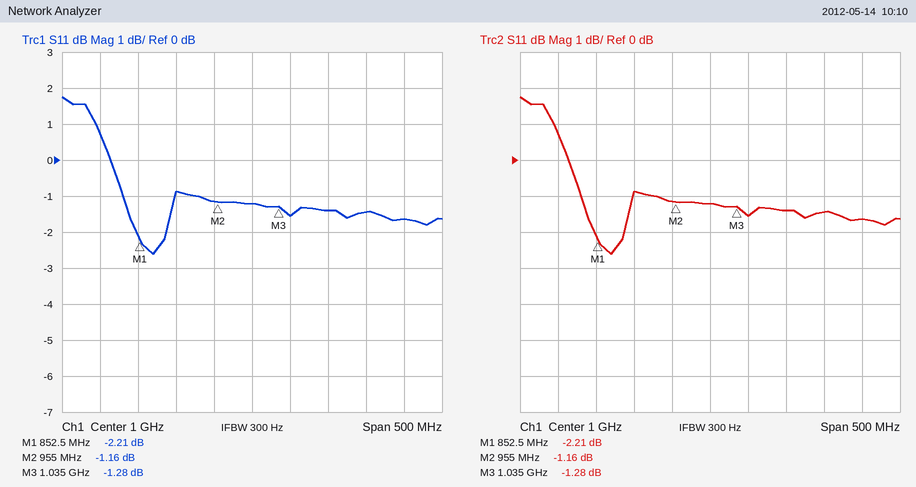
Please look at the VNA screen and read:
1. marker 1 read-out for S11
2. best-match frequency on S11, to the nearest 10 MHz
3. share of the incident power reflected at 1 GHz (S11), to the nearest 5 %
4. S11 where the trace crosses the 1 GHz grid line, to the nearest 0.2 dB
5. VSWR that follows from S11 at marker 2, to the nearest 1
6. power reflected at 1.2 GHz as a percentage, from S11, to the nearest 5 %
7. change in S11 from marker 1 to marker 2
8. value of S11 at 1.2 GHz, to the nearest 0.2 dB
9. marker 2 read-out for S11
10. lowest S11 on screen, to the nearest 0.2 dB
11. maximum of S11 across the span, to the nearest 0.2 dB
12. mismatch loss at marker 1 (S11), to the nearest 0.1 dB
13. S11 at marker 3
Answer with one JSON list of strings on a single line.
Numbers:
["-2.21 dB", "870 MHz", "75 %", "-1.2 dB", "15", "70 %", "1.05 dB", "-1.6 dB", "-1.16 dB", "-2.6 dB", "1.8 dB", "4.0 dB", "-1.28 dB"]
